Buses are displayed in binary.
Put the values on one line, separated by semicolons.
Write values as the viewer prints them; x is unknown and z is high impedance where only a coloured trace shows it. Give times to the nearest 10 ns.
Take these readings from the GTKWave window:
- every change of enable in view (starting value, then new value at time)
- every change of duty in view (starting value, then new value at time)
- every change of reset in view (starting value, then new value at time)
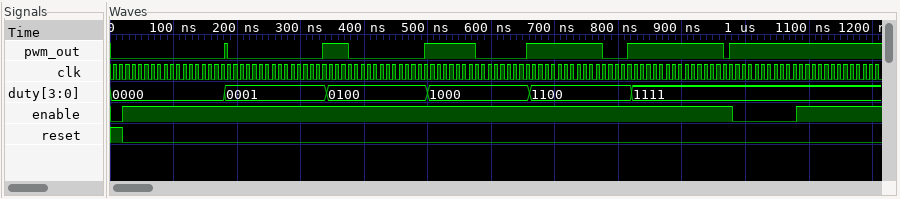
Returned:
0, 1 at 20 ns, 0 at 980 ns, 1 at 1080 ns; 0000, 0001 at 180 ns, 0100 at 340 ns, 1000 at 500 ns, 1100 at 660 ns, 1111 at 820 ns; 1, 0 at 20 ns
